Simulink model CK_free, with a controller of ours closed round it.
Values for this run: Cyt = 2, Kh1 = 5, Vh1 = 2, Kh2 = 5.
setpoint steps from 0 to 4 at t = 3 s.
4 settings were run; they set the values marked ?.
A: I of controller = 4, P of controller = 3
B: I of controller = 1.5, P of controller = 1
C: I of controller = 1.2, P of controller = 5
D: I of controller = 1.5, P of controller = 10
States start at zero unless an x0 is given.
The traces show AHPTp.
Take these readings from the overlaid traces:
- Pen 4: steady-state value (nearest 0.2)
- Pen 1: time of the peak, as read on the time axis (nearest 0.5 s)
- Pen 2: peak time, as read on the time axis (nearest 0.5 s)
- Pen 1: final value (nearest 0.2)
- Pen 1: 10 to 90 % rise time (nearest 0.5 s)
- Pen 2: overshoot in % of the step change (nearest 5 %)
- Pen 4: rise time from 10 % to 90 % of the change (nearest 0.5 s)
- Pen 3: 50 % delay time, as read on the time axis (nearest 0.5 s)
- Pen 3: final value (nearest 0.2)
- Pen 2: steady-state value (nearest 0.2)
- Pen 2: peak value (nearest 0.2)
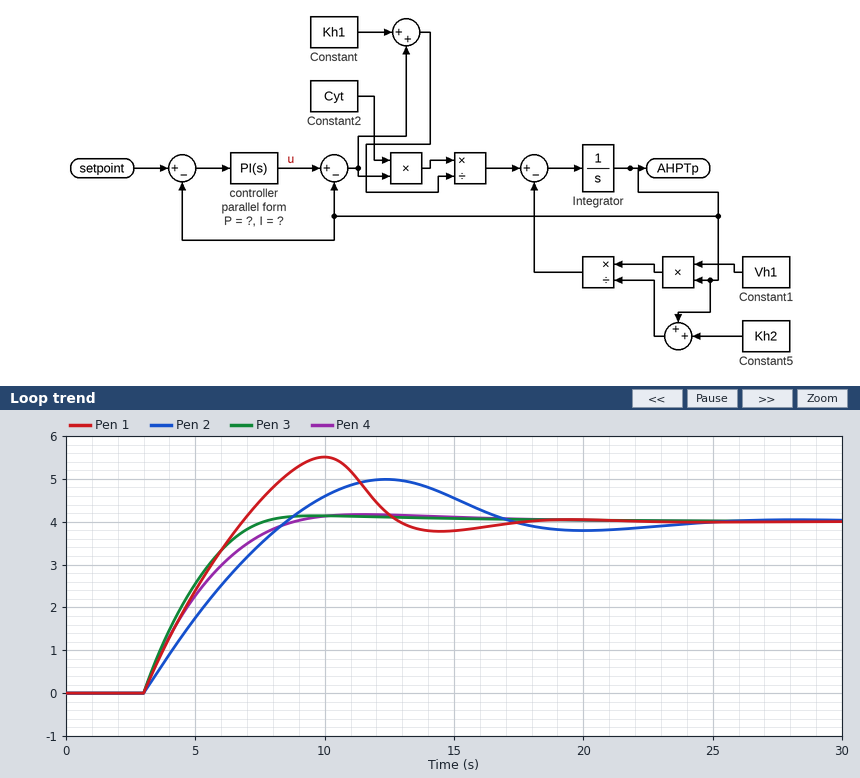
4.0
10.0 s
12.5 s
4.0
3.0 s
25 %
4.0 s
4.5 s
4.0
4.0
5.0
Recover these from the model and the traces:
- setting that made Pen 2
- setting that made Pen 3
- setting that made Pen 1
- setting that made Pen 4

B
D
A
C
